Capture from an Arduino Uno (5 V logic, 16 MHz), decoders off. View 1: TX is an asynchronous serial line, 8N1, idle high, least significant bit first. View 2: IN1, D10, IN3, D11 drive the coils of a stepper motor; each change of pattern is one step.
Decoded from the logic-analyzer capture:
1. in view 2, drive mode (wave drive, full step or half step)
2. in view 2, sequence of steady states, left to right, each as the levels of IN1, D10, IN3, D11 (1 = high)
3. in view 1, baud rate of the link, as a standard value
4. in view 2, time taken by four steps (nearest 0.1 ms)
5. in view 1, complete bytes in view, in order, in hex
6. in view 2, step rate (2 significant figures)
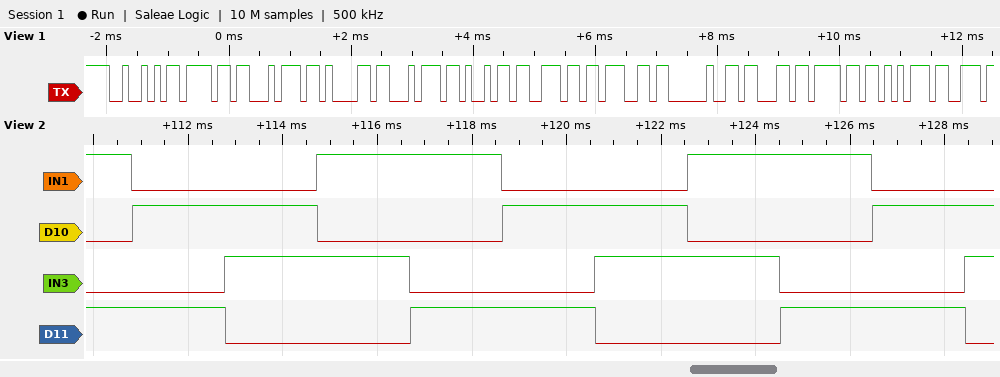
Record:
full step
1001 0101 0110 1010 1001 0101 0110 1010 1001 0101 0110
9600 baud
7.8 ms
52 6F 74 61 74 69 6E 67 20 63 6F 75
510 steps/s
